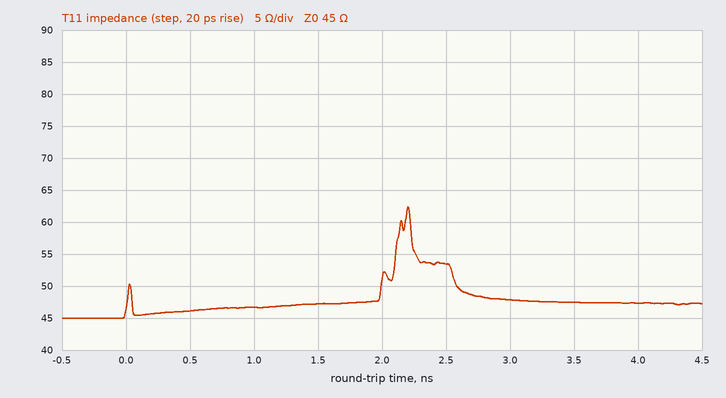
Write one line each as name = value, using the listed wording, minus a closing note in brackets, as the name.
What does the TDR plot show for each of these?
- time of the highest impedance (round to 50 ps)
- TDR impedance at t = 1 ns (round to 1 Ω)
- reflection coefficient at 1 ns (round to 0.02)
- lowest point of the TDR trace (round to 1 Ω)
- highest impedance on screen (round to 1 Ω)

time of the highest impedance = 2.20 ns
TDR impedance at t = 1 ns = 47 Ω
reflection coefficient at 1 ns = +0.02
lowest point of the TDR trace = 45 Ω
highest impedance on screen = 62 Ω
